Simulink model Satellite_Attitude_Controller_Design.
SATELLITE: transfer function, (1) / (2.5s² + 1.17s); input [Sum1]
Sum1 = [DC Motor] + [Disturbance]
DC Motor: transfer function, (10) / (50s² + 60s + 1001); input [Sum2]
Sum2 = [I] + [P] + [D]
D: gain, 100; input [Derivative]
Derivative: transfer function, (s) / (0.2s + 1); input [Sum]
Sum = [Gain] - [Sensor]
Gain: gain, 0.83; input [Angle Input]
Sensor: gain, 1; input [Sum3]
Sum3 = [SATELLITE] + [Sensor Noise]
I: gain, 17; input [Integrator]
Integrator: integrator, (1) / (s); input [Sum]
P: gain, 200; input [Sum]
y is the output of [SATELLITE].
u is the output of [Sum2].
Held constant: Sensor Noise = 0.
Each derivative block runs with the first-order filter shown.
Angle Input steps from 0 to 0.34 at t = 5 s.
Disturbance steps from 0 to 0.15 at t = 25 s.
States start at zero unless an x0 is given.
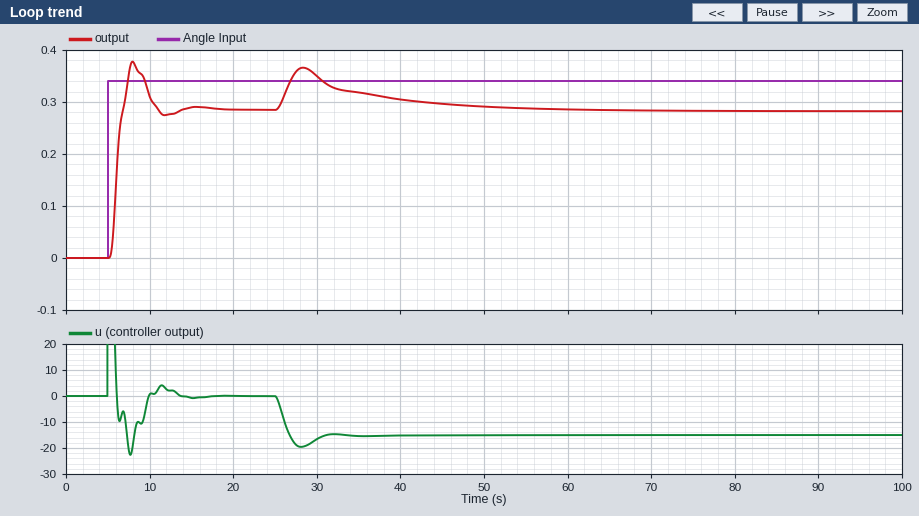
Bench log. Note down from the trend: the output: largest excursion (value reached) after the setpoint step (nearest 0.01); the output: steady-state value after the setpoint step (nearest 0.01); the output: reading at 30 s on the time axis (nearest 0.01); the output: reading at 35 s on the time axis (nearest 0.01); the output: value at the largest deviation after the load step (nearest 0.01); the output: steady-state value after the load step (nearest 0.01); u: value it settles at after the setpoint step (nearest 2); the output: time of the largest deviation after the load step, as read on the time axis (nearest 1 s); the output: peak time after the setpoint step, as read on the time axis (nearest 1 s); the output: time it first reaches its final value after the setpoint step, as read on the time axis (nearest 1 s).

0.38
0.28
0.35
0.32
0.37
0.28
0
28 s
8 s
7 s
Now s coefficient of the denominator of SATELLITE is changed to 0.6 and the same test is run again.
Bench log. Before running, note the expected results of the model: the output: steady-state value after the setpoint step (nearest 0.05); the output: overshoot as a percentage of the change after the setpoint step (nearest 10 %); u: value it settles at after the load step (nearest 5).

0.30
50 %
-15
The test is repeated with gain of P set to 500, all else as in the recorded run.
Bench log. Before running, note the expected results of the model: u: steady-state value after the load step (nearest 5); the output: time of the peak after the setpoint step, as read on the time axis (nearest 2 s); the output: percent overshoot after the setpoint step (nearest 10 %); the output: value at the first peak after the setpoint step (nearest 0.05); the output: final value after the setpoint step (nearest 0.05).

-15
6 s
60 %
0.45
0.30
